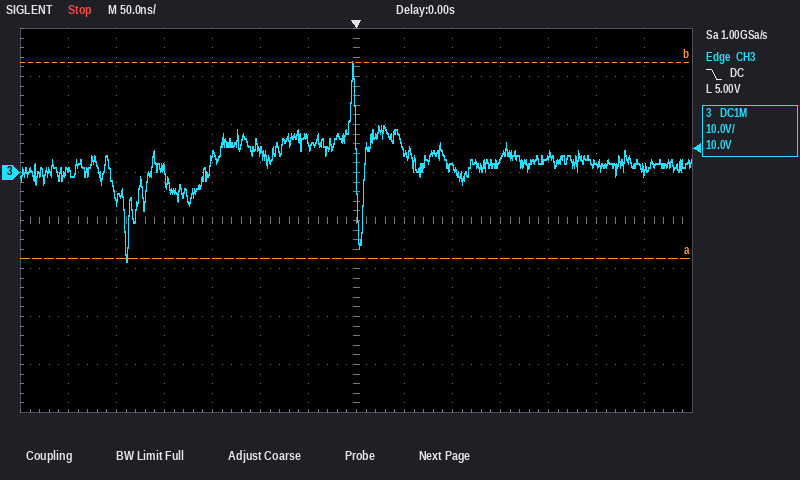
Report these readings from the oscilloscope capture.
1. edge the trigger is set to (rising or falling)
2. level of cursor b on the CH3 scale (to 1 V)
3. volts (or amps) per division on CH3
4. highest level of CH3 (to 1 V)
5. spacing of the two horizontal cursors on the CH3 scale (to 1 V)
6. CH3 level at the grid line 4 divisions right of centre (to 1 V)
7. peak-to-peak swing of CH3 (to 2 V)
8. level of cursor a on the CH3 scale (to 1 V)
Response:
falling
23 V
10 V
23 V
41 V
4 V
42 V
-18 V
